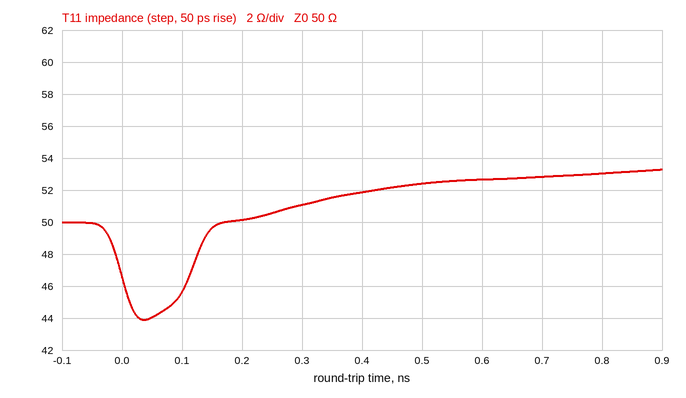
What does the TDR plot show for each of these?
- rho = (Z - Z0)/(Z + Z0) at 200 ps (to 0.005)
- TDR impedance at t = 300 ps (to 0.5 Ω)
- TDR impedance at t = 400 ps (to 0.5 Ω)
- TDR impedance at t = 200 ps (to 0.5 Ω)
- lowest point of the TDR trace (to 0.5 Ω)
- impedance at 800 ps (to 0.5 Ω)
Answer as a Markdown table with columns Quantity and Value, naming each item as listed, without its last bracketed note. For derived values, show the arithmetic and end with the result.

| Quantity | Value |
|---|---|
| rho = (Z - Z0)/(Z + Z0) at 200 ps | (50 − 50)/(50 + 50) ≈ 0.000 |
| TDR impedance at t = 300 ps | 51.0 Ω |
| TDR impedance at t = 400 ps | 52.0 Ω |
| TDR impedance at t = 200 ps | 50.0 Ω |
| lowest point of the TDR trace | 44.0 Ω |
| impedance at 800 ps | 53.0 Ω |
